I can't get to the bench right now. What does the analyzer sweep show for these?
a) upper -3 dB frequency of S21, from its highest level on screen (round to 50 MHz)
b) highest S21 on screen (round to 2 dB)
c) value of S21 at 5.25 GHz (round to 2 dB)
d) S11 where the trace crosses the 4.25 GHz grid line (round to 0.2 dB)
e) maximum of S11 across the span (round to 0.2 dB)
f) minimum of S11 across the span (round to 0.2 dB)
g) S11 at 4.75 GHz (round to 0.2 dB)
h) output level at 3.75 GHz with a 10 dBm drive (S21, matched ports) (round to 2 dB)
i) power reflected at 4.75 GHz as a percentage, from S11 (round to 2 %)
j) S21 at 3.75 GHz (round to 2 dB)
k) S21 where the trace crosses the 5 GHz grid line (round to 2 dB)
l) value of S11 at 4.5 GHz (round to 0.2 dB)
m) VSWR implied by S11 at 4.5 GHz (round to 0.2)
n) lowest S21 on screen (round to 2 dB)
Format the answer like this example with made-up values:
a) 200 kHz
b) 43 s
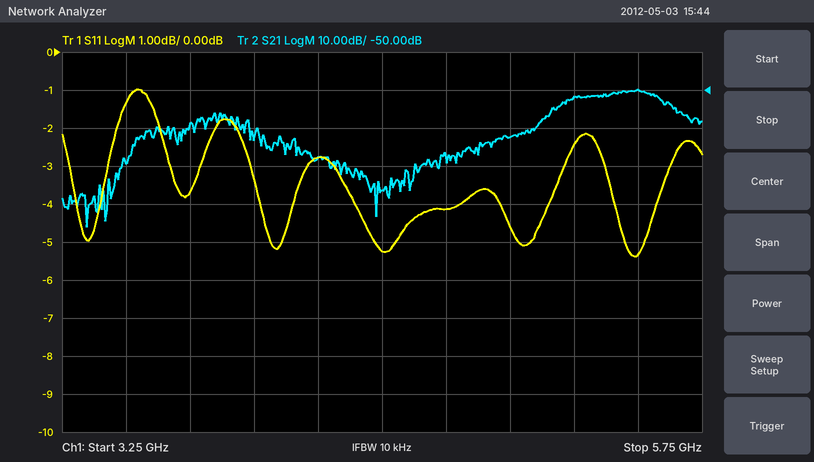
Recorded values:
a) 5.60 GHz
b) -50 dB
c) -52 dB
d) -2.8 dB
e) -1.0 dB
f) -5.4 dB
g) -4.2 dB
h) -50 dBm
i) 38 %
j) -60 dB
k) -62 dB
l) -5.2 dB
m) 3.4
n) -86 dB
